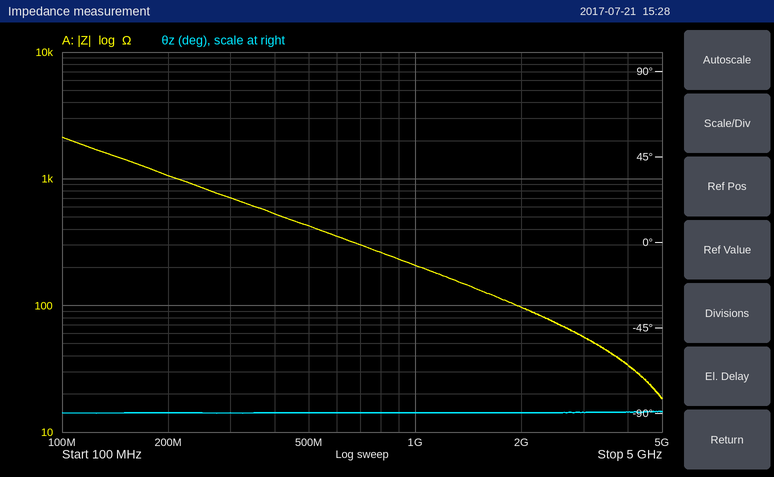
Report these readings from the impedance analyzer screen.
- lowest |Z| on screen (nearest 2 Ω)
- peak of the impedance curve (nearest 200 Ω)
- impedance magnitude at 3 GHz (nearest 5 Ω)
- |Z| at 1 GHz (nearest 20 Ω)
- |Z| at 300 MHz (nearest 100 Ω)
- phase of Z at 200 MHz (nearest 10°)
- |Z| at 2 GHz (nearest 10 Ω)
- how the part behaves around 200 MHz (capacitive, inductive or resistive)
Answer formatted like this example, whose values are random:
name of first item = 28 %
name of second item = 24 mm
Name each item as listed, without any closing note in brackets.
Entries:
lowest |Z| on screen = 18 Ω
peak of the impedance curve = 2.2 kΩ
impedance magnitude at 3 GHz = 55 Ω
|Z| at 1 GHz = 200 Ω
|Z| at 300 MHz = 700 Ω
phase of Z at 200 MHz = -90°
|Z| at 2 GHz = 100 Ω
how the part behaves around 200 MHz = capacitive
